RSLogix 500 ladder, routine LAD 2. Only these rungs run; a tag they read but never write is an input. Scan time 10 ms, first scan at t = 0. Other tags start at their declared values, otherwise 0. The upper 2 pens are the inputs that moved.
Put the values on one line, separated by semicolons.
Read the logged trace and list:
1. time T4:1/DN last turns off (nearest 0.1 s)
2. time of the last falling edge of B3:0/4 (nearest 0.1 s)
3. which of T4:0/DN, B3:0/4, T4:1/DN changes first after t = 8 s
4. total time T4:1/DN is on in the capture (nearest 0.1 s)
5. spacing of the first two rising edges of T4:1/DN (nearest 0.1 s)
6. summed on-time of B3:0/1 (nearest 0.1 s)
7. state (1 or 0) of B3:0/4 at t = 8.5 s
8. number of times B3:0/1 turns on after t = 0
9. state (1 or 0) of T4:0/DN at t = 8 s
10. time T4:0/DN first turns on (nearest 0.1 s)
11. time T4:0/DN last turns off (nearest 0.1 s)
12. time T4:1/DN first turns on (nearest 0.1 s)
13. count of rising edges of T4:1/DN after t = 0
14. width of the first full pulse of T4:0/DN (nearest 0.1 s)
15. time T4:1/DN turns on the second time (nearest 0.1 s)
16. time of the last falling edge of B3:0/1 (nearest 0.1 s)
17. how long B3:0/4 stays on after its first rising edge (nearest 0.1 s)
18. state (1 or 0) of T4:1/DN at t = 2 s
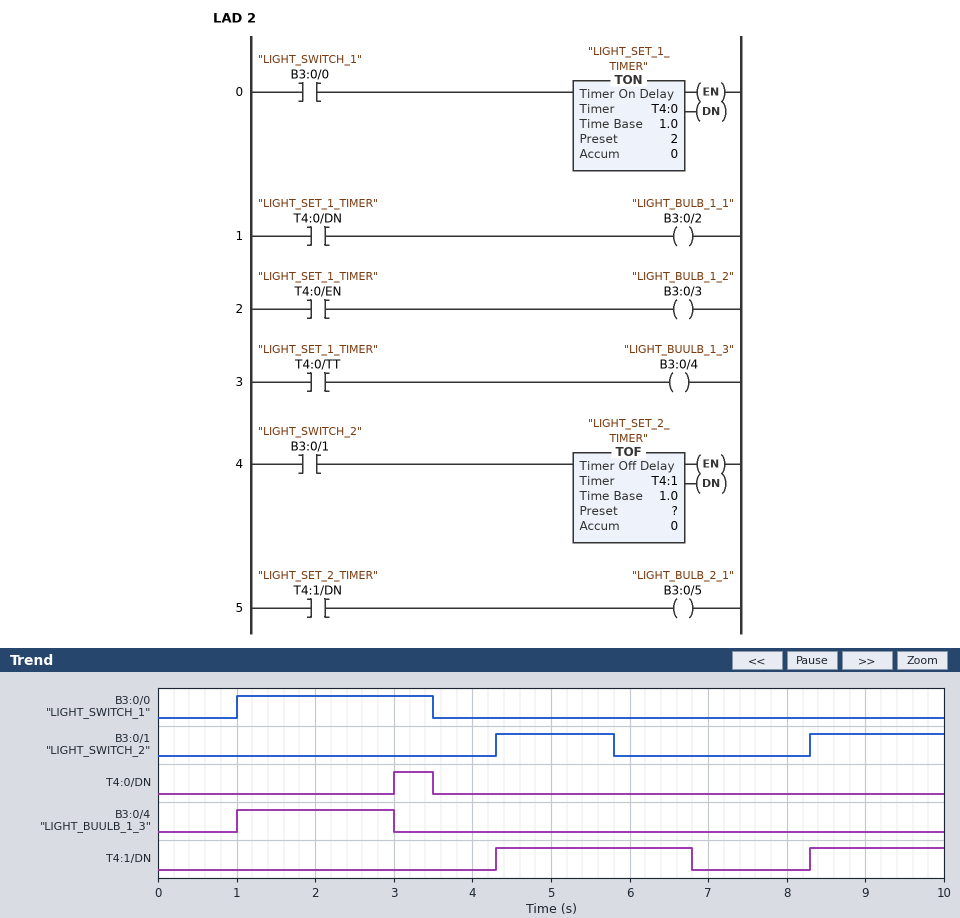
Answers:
6.8 s; 3.0 s; T4:1/DN; 4.2 s; 4.0 s; 3.2 s; 0; 2; 0; 3.0 s; 3.5 s; 4.3 s; 2; 0.5 s; 8.3 s; 5.8 s; 2.0 s; 0
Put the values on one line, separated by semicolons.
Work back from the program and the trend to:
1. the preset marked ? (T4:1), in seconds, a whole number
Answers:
1 s
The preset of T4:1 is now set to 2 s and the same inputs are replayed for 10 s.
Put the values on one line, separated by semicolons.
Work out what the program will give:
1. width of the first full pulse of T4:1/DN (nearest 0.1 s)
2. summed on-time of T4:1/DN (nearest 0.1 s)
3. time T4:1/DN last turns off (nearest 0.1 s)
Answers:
3.5 s; 5.2 s; 7.8 s
